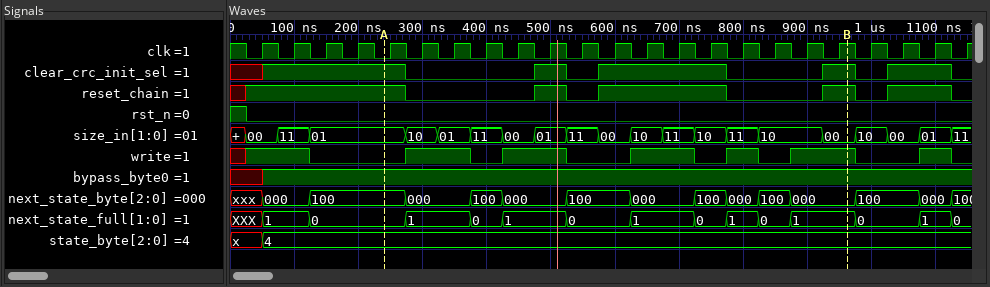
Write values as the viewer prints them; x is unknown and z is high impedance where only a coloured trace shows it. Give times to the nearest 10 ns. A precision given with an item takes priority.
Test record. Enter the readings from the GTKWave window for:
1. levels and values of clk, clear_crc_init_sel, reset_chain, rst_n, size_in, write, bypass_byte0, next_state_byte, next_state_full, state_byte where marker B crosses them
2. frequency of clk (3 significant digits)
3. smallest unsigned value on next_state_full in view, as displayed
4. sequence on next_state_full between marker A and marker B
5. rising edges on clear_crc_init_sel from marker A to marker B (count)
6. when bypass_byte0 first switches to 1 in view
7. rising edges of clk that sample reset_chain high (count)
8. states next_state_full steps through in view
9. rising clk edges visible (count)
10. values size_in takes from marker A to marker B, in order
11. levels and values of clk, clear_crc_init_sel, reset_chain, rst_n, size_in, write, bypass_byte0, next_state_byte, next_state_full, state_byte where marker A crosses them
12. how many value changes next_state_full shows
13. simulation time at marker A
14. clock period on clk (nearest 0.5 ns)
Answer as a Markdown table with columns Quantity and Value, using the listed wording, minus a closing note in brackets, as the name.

| Quantity | Value |
|---|---|
| levels and values of clk, clear_crc_init_sel, reset_chain, rst_n, size_in, write, bypass_byte0, next_state_byte, next_state_full, state_byte where marker B crosses them | clk=1, clear_crc_init_sel=1, reset_chain=1, rst_n=0, size_in=00, write=1, bypass_byte0=1, next_state_byte=000, next_state_full=1, state_byte=4 |
| frequency of clk | 20.0 MHz |
| smallest unsigned value on next_state_full in view, as displayed | 0 |
| sequence on next_state_full between marker A and marker B | 0, 1, 0, 1, 0, 1, 0, 1, 0, 1 |
| rising edges on clear_crc_init_sel from marker A to marker B | 3 |
| when bypass_byte0 first switches to 1 in view | 50 ns |
| rising edges of clk that sample reset_chain high | 13 |
| states next_state_full steps through in view | XXX, 1, 0, 1, 0, 1, 0, 1, 0, 1, 0, 1, 0, 1, 0 |
| rising clk edges visible | 23 |
| values size_in takes from marker A to marker B, in order | 01, 10, 01, 11, 00, 01, 11, 00, 10, 11, 10, 11, 10, 00 |
| levels and values of clk, clear_crc_init_sel, reset_chain, rst_n, size_in, write, bypass_byte0, next_state_byte, next_state_full, state_byte where marker A crosses them | clk=0, clear_crc_init_sel=1, reset_chain=1, rst_n=0, size_in=01, write=0, bypass_byte0=1, next_state_byte=100, next_state_full=0, state_byte=4 |
| how many value changes next_state_full shows | 14 |
| simulation time at marker A | 240 ns |
| clock period on clk | 50 ns |
